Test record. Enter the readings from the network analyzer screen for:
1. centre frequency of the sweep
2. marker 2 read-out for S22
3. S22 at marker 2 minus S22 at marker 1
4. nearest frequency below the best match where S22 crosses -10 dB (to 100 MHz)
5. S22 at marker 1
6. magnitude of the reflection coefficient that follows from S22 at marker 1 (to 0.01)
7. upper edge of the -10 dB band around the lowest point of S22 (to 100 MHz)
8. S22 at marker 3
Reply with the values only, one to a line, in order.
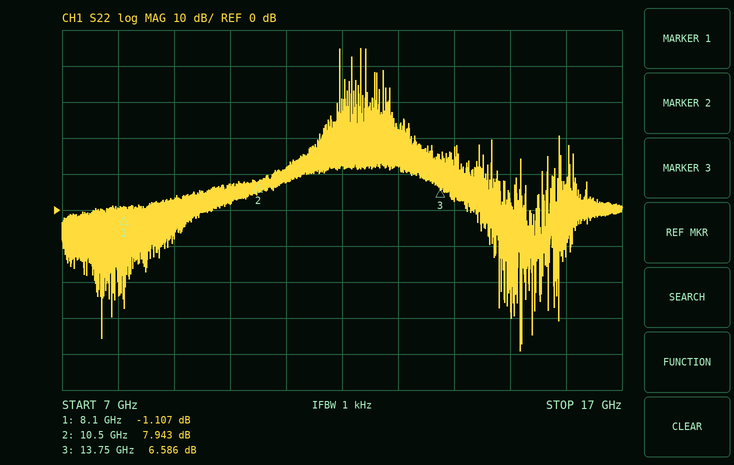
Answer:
12 GHz
7.943 dB
9.050 dB
15.2 GHz
-1.107 dB
0.88
15.2 GHz
6.586 dB
